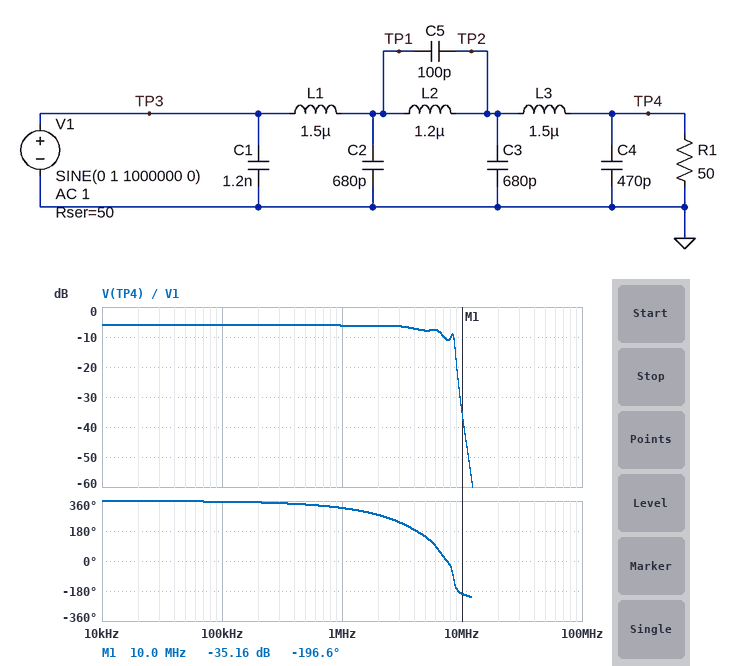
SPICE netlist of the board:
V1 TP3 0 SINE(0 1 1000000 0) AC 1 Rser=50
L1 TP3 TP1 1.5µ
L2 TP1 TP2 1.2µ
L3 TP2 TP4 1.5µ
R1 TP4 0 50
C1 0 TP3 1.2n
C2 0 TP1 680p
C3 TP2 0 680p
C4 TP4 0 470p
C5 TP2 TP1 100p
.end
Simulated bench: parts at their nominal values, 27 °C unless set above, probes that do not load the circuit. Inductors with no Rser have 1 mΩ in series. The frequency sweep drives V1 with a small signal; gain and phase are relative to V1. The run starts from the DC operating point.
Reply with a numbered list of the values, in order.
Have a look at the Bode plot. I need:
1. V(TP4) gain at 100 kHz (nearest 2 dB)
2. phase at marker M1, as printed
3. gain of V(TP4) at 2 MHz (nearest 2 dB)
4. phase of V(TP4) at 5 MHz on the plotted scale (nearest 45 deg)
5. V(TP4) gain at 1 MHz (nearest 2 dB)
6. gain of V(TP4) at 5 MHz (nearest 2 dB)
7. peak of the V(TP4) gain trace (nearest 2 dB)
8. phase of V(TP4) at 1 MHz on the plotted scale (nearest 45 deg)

1. -6 dB
2. -196.6 deg
3. -6 dB
4. 135 deg
5. -6 dB
6. -8 dB
7. -6 dB
8. 315 deg
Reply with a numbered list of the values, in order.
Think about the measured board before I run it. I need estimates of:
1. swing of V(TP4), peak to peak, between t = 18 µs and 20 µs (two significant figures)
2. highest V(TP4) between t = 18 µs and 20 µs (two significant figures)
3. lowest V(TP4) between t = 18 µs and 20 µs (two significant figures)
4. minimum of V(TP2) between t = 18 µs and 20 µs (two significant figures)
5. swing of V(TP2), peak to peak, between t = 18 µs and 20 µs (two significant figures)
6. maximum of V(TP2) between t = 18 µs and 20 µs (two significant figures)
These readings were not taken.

1. 980 mV
2. 490 mV
3. -490 mV
4. -490 mV
5. 970 mV
6. 490 mV
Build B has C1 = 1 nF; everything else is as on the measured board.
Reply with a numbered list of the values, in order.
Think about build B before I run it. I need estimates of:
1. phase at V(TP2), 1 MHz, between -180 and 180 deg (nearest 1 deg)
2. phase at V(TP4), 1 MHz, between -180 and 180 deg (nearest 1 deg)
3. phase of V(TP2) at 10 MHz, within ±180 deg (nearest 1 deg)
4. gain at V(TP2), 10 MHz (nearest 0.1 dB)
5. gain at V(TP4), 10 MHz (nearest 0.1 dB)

1. -29 deg
2. -40 deg
3. -59 deg
4. -25.1 dB
5. -33.4 dB
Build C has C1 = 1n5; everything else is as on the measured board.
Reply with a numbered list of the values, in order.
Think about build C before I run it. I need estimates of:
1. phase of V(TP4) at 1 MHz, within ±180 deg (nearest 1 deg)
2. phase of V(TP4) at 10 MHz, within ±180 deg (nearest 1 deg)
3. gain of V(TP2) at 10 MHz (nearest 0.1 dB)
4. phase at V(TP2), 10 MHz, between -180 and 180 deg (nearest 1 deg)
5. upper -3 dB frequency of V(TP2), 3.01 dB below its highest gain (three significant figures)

1. -44 deg
2. 159 deg
3. -29.1 dB
4. -67 deg
5. 8.66 MHz
